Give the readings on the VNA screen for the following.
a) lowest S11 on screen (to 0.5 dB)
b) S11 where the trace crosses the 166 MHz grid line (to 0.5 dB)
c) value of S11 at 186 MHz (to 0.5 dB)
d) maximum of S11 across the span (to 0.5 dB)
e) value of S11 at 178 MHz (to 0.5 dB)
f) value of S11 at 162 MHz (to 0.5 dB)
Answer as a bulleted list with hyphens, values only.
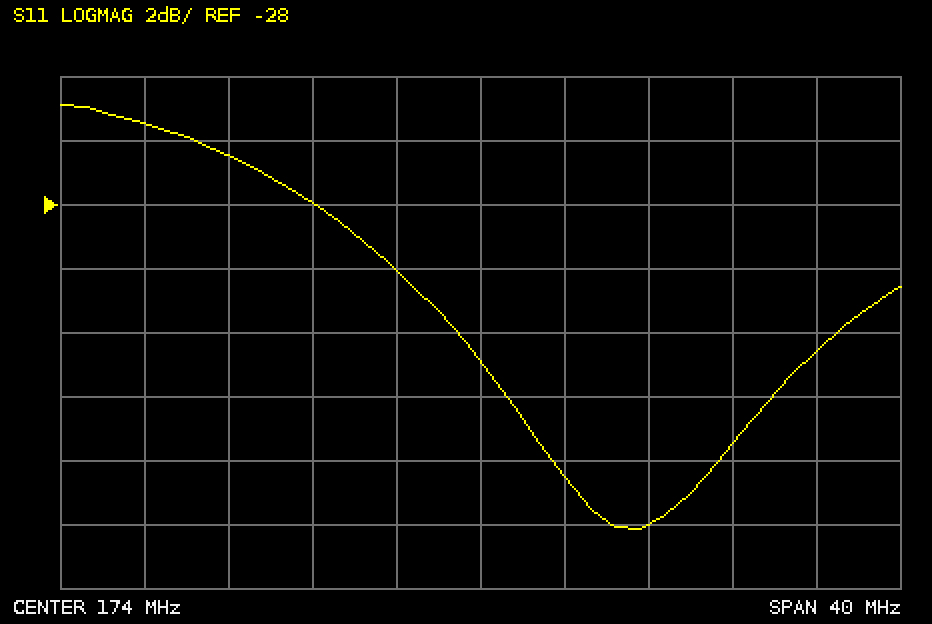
- -38.0 dB
- -28.0 dB
- -35.5 dB
- -25.0 dB
- -36.5 dB
- -26.5 dB
